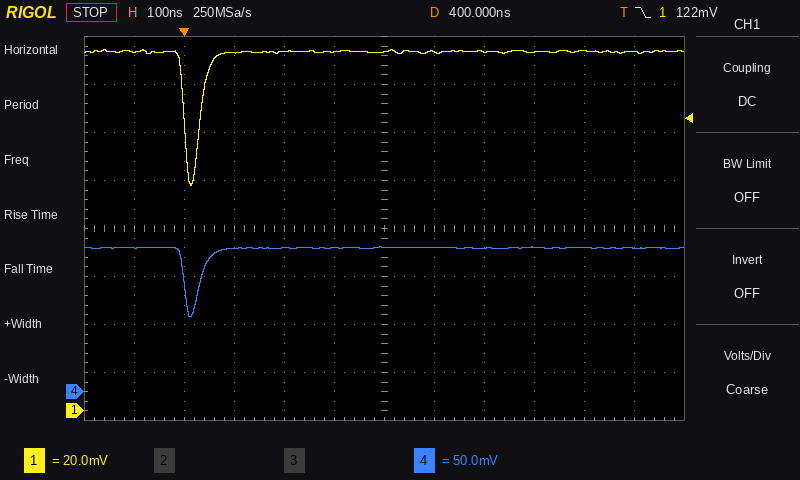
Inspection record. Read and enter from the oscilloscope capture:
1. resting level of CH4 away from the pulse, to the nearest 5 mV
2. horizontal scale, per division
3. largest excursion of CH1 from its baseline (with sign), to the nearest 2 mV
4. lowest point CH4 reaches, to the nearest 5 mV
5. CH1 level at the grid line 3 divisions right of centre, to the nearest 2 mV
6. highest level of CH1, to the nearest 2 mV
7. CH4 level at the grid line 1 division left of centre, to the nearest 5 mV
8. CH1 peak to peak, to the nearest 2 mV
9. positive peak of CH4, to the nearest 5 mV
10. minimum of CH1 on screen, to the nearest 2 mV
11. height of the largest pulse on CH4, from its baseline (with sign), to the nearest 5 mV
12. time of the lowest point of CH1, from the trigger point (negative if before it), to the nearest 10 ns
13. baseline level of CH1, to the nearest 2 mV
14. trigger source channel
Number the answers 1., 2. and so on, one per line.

1. 150 mV
2. 100 ns
3. -56 mV
4. 80 mV
5. 150 mV
6. 150 mV
7. 150 mV
8. 56 mV
9. 150 mV
10. 94 mV
11. -70 mV
12. +10 ns
13. 150 mV
14. CH1
